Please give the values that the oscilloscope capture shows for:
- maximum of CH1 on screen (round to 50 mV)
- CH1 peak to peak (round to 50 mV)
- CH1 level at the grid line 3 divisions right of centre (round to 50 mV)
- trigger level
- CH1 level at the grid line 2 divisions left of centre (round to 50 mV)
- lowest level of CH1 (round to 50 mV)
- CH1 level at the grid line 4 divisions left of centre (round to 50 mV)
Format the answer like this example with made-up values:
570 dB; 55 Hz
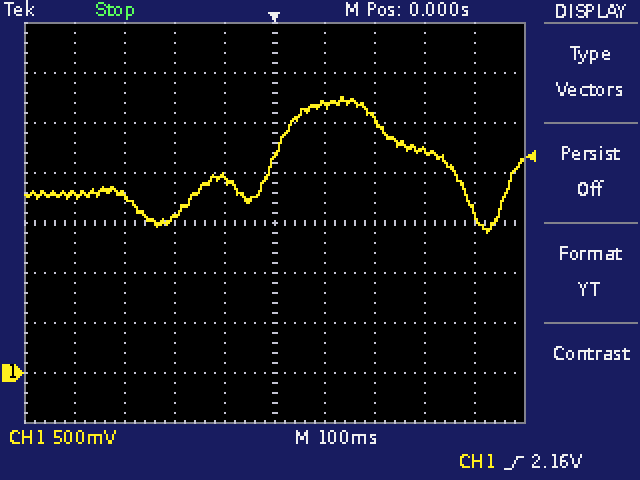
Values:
2.75 V; 1.35 V; 2.20 V; 2.16 V; 1.55 V; 1.40 V; 1.80 V
